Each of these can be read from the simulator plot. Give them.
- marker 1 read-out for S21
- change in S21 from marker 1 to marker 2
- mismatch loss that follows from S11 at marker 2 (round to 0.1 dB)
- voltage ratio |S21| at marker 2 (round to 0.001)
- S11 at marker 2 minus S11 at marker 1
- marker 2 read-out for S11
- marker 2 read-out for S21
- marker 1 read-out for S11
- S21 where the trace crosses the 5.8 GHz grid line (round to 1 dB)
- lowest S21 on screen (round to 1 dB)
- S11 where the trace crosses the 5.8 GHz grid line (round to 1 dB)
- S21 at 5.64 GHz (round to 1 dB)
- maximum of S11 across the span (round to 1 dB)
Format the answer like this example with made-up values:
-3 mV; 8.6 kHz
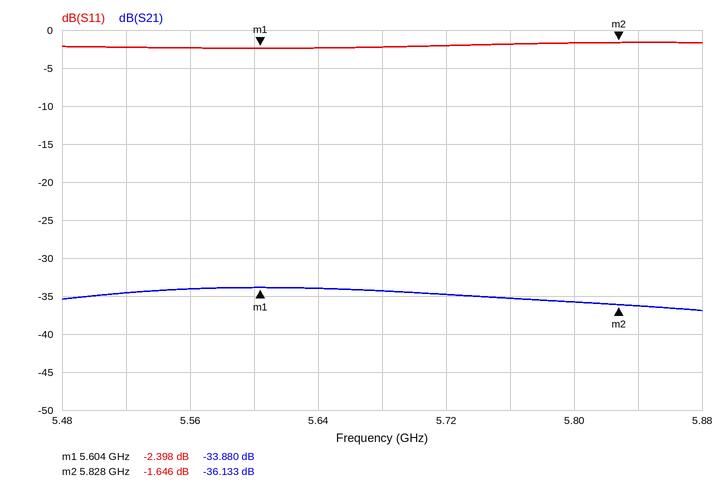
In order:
-33.880 dB; -2.253 dB; 5.0 dB; 0.016; 0.752 dB; -1.646 dB; -36.133 dB; -2.398 dB; -36 dB; -37 dB; -2 dB; -34 dB; -2 dB
